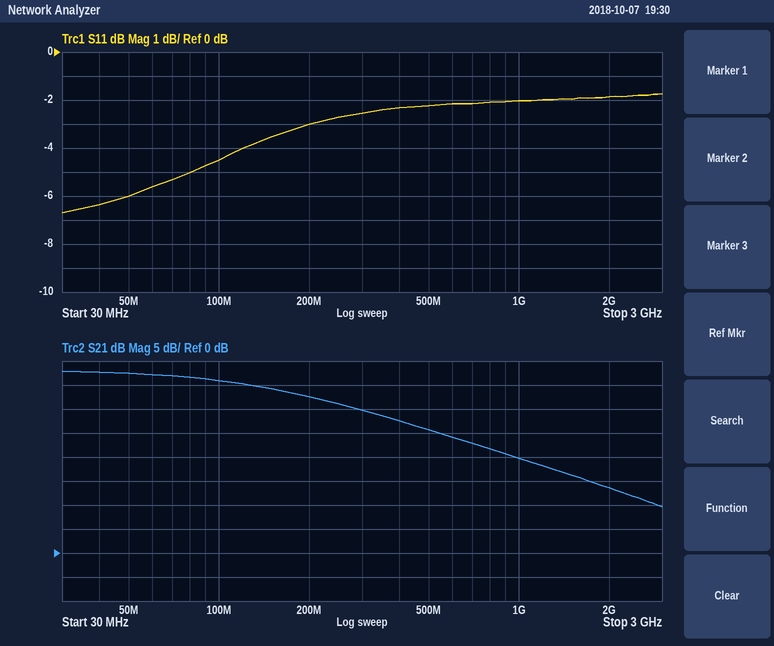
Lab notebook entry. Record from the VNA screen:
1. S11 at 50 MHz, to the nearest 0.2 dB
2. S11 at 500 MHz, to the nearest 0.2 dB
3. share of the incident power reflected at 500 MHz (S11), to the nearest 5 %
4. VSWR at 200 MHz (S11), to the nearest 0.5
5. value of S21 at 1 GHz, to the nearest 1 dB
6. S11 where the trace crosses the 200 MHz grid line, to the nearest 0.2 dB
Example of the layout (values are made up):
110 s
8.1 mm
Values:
-6.0 dB
-2.2 dB
60 %
6.0
20 dB
-3.0 dB
